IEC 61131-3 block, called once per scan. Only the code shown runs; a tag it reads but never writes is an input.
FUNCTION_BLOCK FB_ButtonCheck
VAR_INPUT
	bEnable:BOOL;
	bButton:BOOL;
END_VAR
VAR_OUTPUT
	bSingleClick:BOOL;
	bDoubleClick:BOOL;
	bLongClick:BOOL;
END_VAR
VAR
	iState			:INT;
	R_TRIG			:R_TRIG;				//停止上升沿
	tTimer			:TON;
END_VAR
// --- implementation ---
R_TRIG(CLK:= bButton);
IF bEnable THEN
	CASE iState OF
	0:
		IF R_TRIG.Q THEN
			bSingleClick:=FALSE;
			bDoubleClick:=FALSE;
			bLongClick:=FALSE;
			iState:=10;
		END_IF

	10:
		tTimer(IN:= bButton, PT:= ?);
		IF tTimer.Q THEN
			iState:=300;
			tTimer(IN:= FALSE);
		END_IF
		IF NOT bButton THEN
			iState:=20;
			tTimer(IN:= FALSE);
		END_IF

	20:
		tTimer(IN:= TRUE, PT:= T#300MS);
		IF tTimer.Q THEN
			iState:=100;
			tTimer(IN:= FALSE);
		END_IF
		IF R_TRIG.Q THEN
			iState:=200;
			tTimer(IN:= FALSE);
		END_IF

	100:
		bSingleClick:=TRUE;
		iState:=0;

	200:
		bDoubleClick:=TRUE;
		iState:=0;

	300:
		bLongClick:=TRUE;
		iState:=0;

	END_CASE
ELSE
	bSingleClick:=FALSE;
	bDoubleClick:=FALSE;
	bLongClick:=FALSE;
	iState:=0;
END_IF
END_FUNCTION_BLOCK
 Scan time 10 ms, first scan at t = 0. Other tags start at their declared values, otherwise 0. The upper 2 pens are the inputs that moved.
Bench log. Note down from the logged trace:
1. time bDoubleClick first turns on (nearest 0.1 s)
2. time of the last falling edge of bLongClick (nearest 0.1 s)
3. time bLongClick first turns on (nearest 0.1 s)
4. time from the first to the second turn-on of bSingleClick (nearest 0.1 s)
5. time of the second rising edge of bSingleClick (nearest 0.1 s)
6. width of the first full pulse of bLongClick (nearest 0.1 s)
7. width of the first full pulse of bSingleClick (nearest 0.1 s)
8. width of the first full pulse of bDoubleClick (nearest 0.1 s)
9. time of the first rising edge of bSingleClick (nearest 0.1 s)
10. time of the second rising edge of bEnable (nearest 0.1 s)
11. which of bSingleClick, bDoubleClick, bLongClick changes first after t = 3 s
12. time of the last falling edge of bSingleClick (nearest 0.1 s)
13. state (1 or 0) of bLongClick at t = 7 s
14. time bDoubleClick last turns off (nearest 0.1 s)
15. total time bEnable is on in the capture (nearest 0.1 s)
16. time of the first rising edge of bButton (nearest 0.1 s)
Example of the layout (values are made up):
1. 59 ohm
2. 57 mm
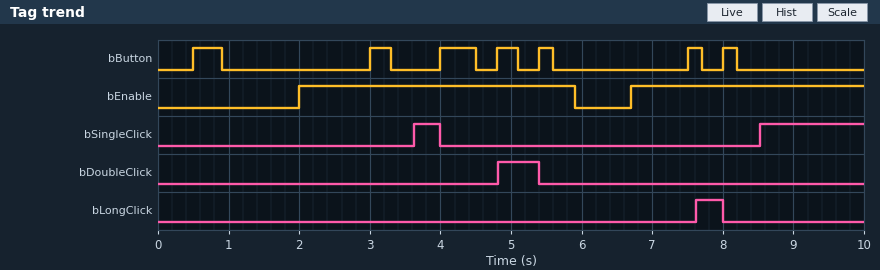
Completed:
1. 4.8 s
2. 8.0 s
3. 7.6 s
4. 4.9 s
5. 8.5 s
6. 0.4 s
7. 0.4 s
8. 0.6 s
9. 3.6 s
10. 6.7 s
11. bSingleClick
12. 4.0 s
13. 0
14. 5.4 s
15. 7.2 s
16. 0.5 s
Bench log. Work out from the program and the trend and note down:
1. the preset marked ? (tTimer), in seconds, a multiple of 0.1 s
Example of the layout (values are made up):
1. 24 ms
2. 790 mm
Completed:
1. 2.0 s
